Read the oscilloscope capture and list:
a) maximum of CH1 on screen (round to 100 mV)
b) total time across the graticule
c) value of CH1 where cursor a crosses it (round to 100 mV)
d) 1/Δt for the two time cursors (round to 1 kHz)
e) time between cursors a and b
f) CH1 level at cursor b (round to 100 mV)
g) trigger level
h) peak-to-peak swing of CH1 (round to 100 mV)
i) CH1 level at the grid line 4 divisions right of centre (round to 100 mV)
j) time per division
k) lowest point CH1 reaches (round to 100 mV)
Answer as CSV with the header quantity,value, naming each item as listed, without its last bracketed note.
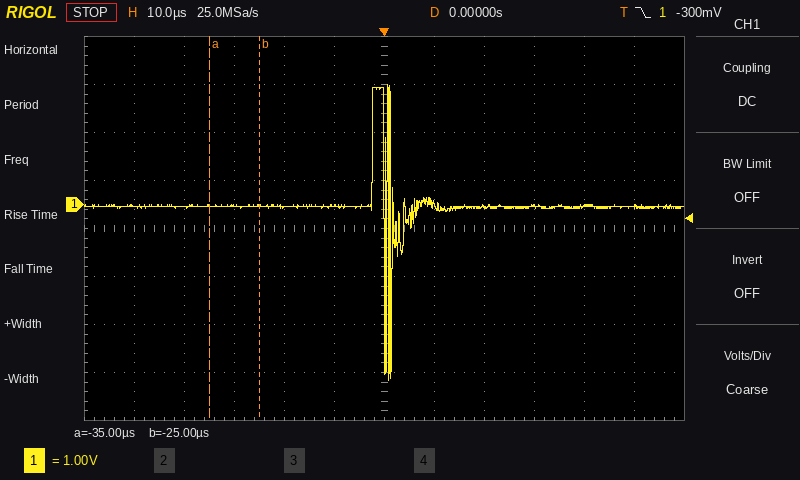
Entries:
quantity,value
maximum of CH1 on screen,2.5 V
total time across the graticule,120 µs
value of CH1 where cursor a crosses it,0.0 V
1/Δt for the two time cursors,100 kHz
time between cursors a and b,10 µs
CH1 level at cursor b,0.0 V
trigger level,-300 mV
peak-to-peak swing of CH1,6.2 V
CH1 level at the grid line 4 divisions right of centre,0.0 V
time per division,10 µs
lowest point CH1 reaches,-3.7 V
